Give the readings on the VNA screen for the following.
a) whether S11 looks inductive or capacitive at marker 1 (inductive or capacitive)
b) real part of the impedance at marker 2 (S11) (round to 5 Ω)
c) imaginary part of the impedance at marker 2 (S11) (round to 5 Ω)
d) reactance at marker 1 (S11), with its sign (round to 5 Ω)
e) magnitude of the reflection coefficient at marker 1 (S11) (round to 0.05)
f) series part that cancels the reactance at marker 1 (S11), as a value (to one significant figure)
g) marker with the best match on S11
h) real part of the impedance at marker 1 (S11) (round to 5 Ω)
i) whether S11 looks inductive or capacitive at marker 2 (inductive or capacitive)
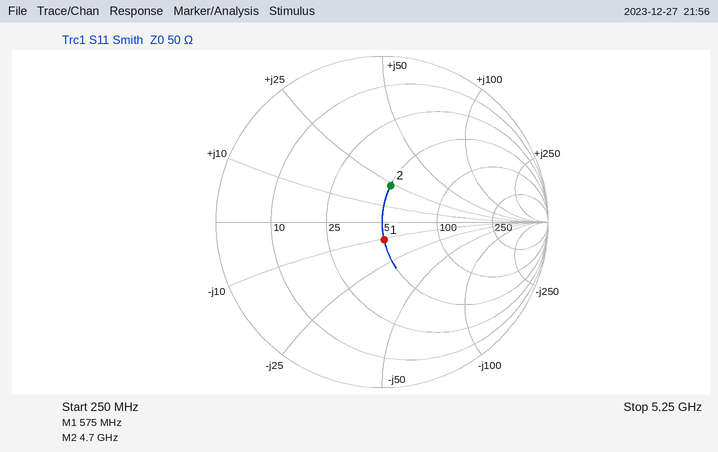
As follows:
capacitive
50 Ω
+25 Ω
-10 Ω
0.10
3 nH
marker 1
50 Ω
inductive
